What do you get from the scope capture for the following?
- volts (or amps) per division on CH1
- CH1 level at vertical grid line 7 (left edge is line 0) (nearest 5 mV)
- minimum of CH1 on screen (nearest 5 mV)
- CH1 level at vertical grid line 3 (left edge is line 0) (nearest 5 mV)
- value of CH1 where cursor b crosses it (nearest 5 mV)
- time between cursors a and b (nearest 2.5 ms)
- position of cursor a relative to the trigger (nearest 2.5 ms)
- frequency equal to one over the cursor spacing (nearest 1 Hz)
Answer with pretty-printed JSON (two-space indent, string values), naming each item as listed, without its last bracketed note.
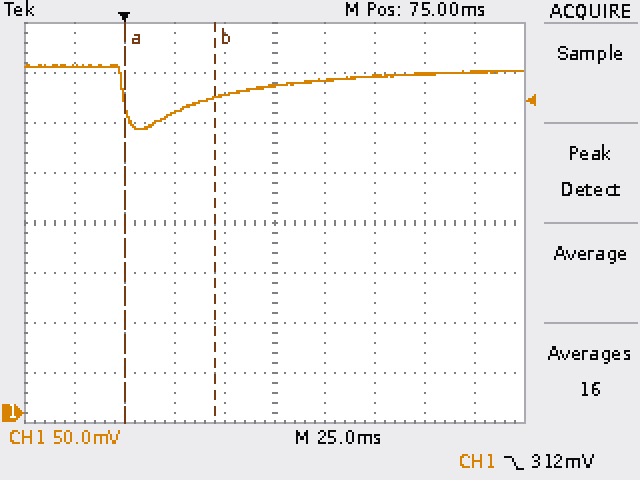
{
  "volts (or amps) per division on CH1": "50 mV",
  "CH1 level at vertical grid line 7 (left edge is line 0)": "335 mV",
  "minimum of CH1 on screen": "285 mV",
  "CH1 level at vertical grid line 3 (left edge is line 0)": "300 mV",
  "value of CH1 where cursor b crosses it": "315 mV",
  "time between cursors a and b": "45.0 ms",
  "position of cursor a relative to the trigger": "0.0 ms",
  "frequency equal to one over the cursor spacing": "22 Hz"
}
